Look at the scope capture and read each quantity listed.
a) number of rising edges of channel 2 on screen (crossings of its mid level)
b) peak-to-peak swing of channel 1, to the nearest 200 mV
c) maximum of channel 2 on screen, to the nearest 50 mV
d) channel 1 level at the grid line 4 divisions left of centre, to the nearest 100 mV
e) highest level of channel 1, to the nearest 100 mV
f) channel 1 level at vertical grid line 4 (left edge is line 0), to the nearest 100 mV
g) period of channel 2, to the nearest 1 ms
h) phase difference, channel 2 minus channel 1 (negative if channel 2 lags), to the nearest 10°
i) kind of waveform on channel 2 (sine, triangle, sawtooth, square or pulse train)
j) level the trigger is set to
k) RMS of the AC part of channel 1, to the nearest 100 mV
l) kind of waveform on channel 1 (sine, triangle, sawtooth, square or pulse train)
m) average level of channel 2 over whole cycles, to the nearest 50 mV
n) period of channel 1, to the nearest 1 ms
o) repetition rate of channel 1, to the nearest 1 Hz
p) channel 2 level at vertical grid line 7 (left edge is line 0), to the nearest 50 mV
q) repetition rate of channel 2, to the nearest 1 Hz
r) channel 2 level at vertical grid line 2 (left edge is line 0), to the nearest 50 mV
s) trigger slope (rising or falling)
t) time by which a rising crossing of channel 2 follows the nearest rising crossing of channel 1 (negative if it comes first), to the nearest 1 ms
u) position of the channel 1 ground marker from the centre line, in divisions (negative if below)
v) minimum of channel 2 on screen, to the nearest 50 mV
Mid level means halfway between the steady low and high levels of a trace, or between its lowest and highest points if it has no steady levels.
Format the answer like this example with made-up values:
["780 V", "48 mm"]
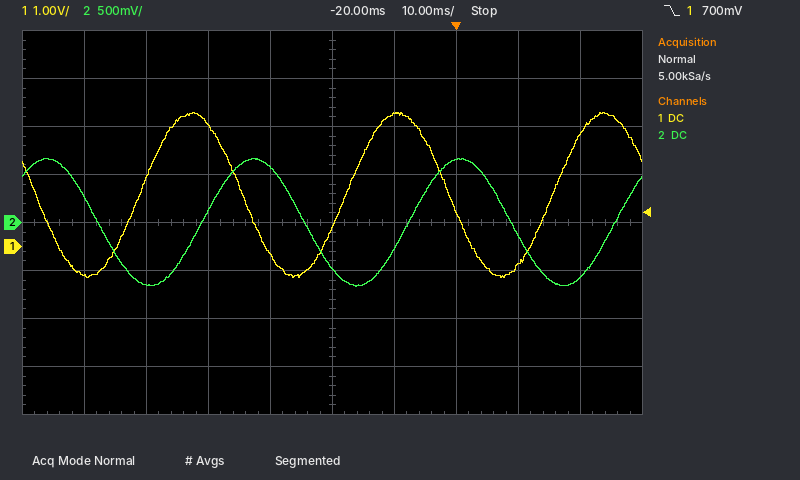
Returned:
["3", "3.4 V", "650 mV", "-600 mV", "2.8 V", "-200 mV", "33 ms", "-110°", "sine", "700 mV", "1.2 V", "sine", "0 mV", "33 ms", "30 Hz", "650 mV", "30 Hz", "-650 mV", "falling", "+10 ms", "-0.5 div", "-650 mV"]
